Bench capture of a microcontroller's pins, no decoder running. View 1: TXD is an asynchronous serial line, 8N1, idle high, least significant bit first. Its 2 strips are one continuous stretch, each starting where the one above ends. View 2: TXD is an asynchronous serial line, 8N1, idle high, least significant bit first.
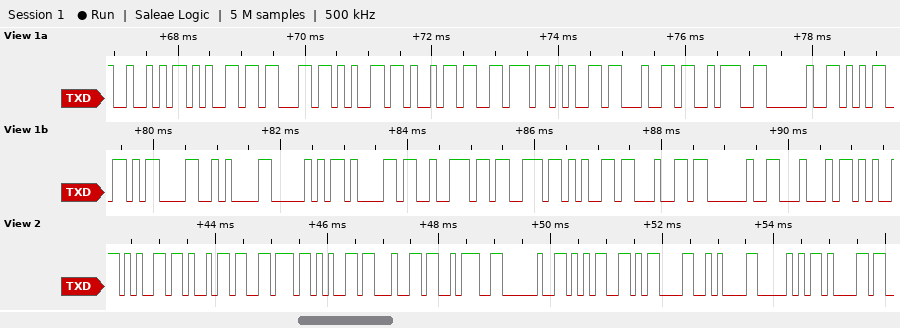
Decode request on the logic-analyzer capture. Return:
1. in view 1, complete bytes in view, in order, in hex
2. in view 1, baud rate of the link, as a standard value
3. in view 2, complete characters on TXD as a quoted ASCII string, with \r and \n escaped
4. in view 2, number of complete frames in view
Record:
52 65 63 65 69 76 65 64 3A 20 35 0D 0A 50 61 72 73 65 64 20 44
9600 baud
"eived: 5\r\nPa"
12
